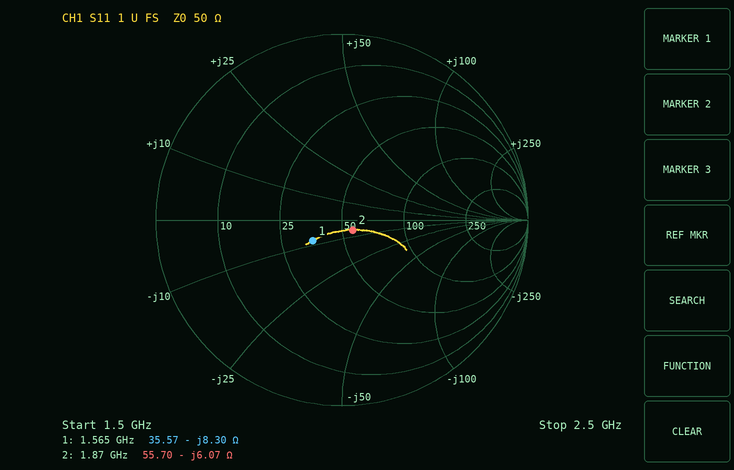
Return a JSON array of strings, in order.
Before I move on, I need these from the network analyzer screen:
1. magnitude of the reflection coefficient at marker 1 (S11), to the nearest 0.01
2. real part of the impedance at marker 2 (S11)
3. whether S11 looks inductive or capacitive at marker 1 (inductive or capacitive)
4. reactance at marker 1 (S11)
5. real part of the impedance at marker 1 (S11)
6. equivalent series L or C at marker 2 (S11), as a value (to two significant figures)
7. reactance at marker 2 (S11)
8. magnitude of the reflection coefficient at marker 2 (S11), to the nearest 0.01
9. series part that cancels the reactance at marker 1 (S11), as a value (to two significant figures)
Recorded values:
["0.19", "55.70 Ω", "capacitive", "-8.30 Ω", "35.57 Ω", "14 pF", "-6.07 Ω", "0.08", "840 pH"]
